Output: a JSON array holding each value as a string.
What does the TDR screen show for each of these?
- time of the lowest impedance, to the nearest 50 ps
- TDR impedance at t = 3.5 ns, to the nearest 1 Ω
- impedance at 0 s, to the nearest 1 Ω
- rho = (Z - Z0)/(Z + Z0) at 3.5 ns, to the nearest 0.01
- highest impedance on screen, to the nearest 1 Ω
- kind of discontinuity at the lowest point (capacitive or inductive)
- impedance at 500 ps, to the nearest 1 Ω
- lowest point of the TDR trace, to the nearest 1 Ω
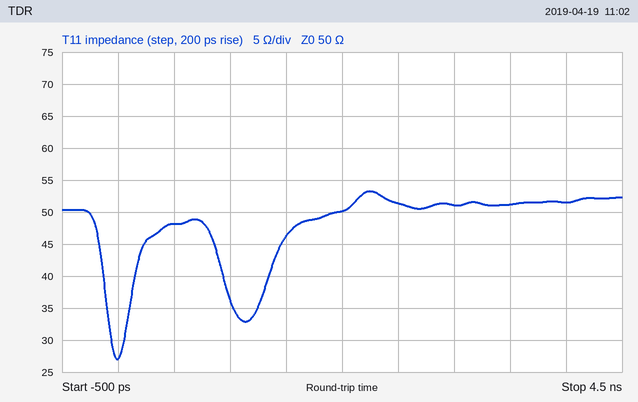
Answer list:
["0 ps", "51 Ω", "27 Ω", "+0.01", "53 Ω", "capacitive", "48 Ω", "27 Ω"]
